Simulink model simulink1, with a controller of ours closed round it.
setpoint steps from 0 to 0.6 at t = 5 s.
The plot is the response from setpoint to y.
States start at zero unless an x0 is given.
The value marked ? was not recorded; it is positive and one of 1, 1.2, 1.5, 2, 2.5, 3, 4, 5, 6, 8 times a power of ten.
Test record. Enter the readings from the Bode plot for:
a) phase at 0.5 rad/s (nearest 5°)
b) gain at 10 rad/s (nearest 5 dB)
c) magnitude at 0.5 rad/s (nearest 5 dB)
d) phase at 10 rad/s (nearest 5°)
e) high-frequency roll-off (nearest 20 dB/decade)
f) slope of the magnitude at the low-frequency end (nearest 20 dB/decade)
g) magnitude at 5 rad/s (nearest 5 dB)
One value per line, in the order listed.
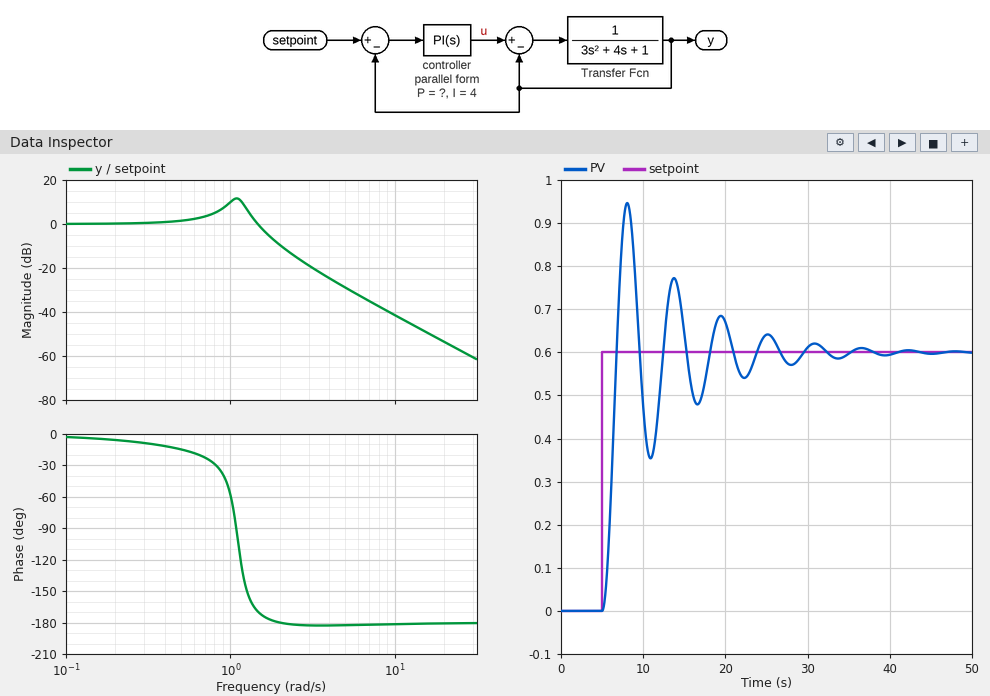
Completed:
-15°
-40 dB
0 dB
-180°
-40 dB/decade
0 dB/decade
-30 dB
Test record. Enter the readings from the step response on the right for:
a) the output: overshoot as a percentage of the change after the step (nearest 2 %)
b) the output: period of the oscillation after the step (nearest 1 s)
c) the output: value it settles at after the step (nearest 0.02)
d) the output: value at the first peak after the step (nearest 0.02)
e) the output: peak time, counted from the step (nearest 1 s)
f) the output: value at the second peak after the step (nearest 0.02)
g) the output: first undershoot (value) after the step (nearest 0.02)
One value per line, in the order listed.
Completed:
58 %
6 s
0.60
0.94
3 s
0.78
0.36
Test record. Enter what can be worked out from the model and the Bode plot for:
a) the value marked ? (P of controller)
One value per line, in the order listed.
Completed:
2.5
